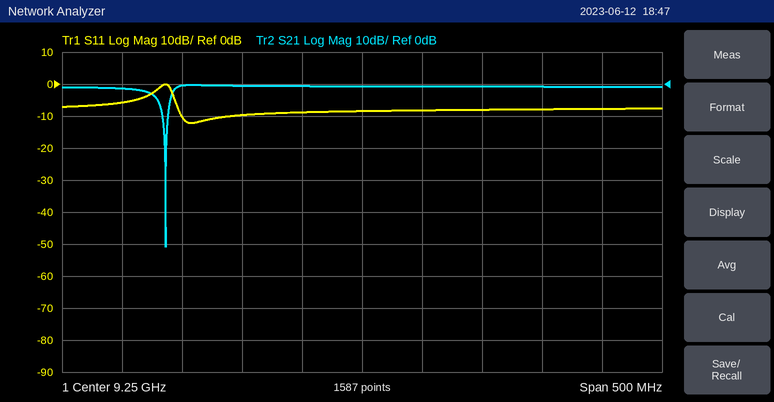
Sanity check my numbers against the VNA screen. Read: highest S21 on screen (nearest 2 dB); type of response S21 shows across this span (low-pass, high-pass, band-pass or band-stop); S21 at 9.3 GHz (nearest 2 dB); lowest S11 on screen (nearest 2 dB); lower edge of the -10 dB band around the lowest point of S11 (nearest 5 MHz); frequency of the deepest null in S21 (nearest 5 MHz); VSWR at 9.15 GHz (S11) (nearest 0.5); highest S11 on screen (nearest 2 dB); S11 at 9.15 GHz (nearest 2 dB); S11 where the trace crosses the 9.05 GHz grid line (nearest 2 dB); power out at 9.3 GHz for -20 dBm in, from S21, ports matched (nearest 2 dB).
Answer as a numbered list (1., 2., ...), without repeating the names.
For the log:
1. 0 dB
2. band-stop
3. 0 dB
4. -12 dB
5. 9.100 GHz
6. 9.085 GHz
7. 2.0
8. 0 dB
9. -10 dB
10. -6 dB
11. -20 dBm
